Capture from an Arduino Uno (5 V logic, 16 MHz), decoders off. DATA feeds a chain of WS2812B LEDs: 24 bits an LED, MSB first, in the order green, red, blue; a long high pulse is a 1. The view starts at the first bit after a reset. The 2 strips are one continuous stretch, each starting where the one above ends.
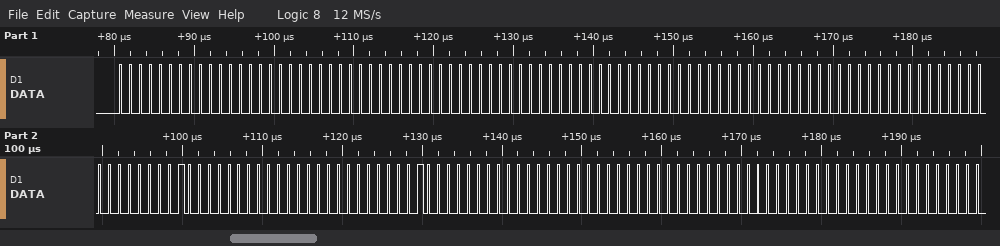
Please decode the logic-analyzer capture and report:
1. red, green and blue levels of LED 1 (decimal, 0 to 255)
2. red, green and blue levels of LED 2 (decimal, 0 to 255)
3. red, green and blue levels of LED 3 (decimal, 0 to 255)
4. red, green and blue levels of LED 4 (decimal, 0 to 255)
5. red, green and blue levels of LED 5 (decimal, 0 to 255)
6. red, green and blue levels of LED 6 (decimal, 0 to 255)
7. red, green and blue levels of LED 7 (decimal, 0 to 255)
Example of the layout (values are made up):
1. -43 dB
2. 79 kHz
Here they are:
1. 0, 0, 0
2. 0, 0, 0
3. 0, 0, 0
4. 0, 0, 1
5. 0, 0, 1
6. 0, 0, 0
7. 0, 0, 0
